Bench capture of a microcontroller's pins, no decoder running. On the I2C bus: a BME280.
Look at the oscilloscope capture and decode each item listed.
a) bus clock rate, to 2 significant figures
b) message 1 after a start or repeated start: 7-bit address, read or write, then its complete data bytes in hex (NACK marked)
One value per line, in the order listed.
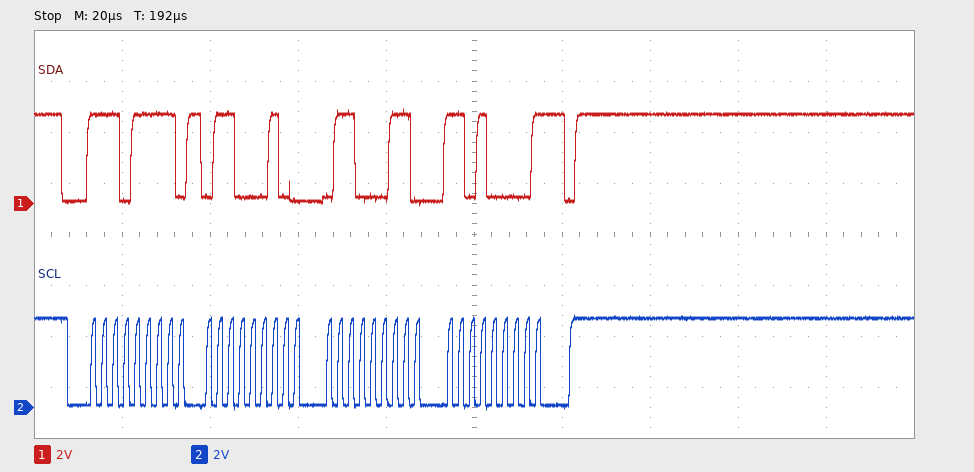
400 kHz
0x77 read: 62 63 D0 NACK
